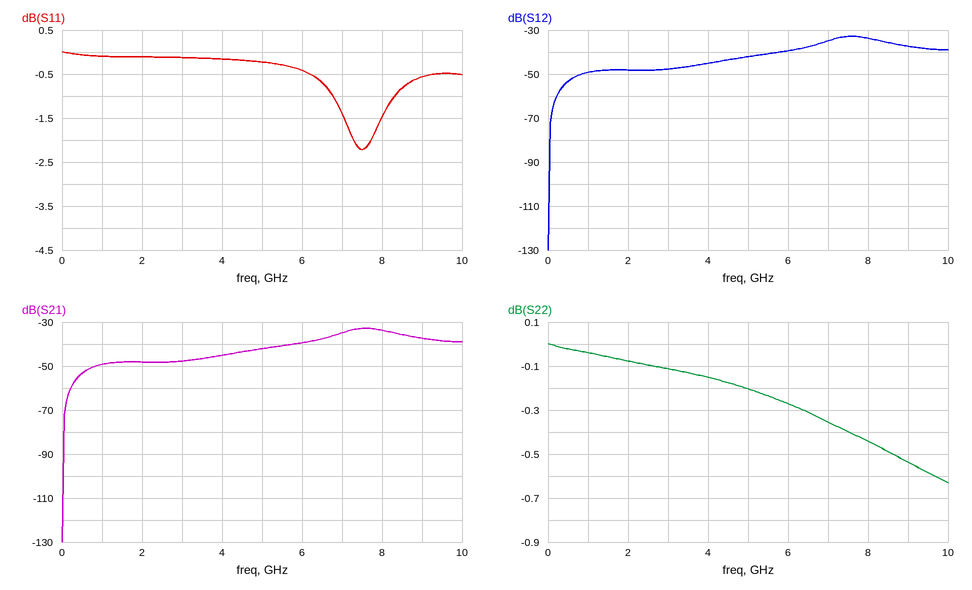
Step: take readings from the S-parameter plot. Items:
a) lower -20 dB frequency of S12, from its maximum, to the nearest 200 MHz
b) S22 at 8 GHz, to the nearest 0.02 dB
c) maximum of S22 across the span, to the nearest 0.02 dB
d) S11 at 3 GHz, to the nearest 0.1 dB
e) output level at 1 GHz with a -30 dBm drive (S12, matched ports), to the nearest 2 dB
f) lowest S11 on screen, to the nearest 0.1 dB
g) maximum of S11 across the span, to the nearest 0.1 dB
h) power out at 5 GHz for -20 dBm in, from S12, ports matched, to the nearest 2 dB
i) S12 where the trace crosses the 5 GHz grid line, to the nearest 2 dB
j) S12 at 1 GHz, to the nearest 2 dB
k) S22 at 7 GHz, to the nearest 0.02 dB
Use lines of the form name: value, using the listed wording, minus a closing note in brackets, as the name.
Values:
lower -20 dB frequency of S12, from its maximum, to the nearest 200 MHz: 600 MHz
S22 at 8 GHz, to the nearest 0.02 dB: -0.44 dB
maximum of S22 across the span, to the nearest 0.02 dB: 0.00 dB
S11 at 3 GHz, to the nearest 0.1 dB: -0.1 dB
output level at 1 GHz with a -30 dBm drive (S12, matched ports), to the nearest 2 dB: -80 dBm
lowest S11 on screen, to the nearest 0.1 dB: -2.2 dB
maximum of S11 across the span, to the nearest 0.1 dB: 0.0 dB
power out at 5 GHz for -20 dBm in, from S12, ports matched, to the nearest 2 dB: -62 dBm
S12 where the trace crosses the 5 GHz grid line, to the nearest 2 dB: -42 dB
S12 at 1 GHz, to the nearest 2 dB: -50 dB
S22 at 7 GHz, to the nearest 0.02 dB: -0.36 dB
